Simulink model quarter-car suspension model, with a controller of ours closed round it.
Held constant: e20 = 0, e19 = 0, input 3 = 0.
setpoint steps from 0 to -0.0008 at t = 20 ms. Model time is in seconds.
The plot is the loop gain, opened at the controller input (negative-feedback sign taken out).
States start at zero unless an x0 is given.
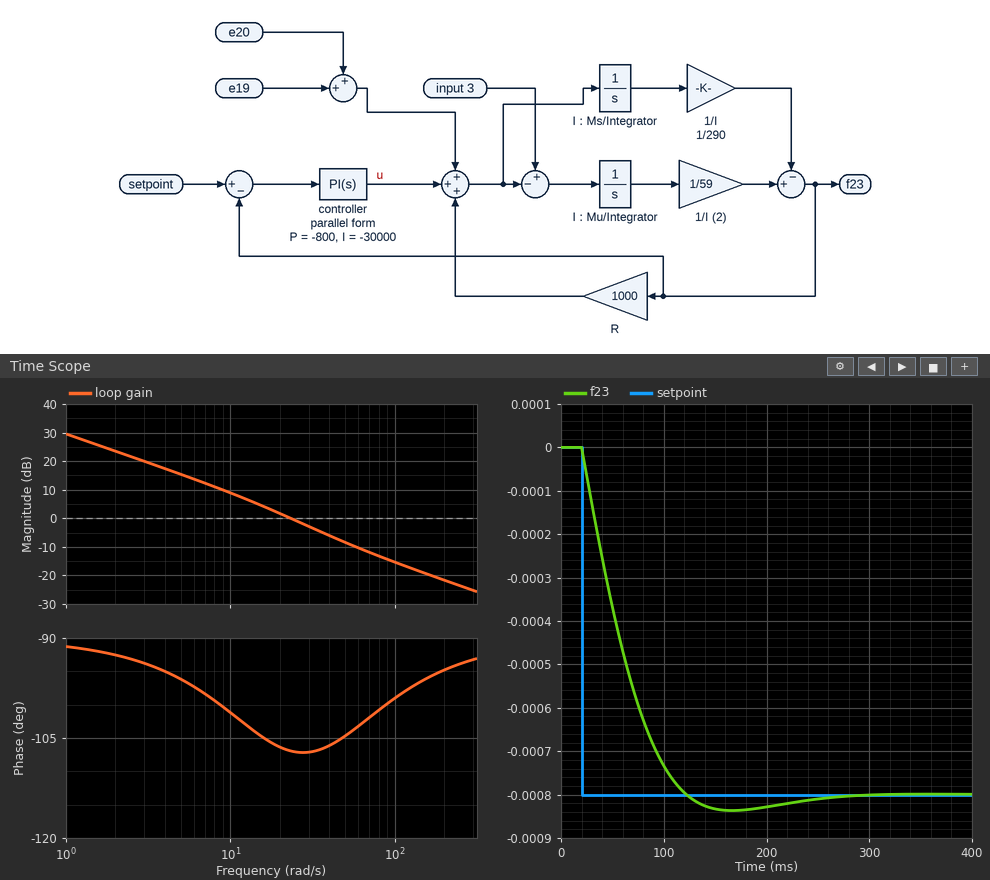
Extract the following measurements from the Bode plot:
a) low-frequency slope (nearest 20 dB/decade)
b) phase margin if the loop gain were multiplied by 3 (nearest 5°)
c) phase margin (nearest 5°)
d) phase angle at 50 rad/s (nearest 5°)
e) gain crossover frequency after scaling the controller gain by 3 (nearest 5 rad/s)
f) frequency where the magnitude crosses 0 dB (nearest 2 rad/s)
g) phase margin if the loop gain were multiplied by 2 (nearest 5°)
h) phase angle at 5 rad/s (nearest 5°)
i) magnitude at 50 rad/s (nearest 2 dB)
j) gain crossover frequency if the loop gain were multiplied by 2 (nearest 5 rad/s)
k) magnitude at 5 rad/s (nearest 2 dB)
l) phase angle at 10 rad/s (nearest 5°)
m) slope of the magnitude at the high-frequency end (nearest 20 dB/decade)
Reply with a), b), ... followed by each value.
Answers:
a) -20 dB/decade
b) 75°
c) 75°
d) -105°
e) 55 rad/s
f) 24 rad/s
g) 75°
h) -95°
i) -8 dB
j) 40 rad/s
k) 16 dB
l) -100°
m) -20 dB/decade
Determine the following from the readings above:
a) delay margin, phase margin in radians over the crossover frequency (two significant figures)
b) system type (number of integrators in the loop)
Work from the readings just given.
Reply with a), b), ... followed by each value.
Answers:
a) 0.055 s
b) 1
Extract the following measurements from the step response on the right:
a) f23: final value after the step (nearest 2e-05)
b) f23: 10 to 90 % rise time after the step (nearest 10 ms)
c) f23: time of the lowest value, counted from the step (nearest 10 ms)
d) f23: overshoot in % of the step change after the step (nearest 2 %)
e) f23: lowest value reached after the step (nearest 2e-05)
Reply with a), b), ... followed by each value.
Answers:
a) -0.00080
b) 70 ms
c) 150 ms
d) 4 %
e) -0.00084
